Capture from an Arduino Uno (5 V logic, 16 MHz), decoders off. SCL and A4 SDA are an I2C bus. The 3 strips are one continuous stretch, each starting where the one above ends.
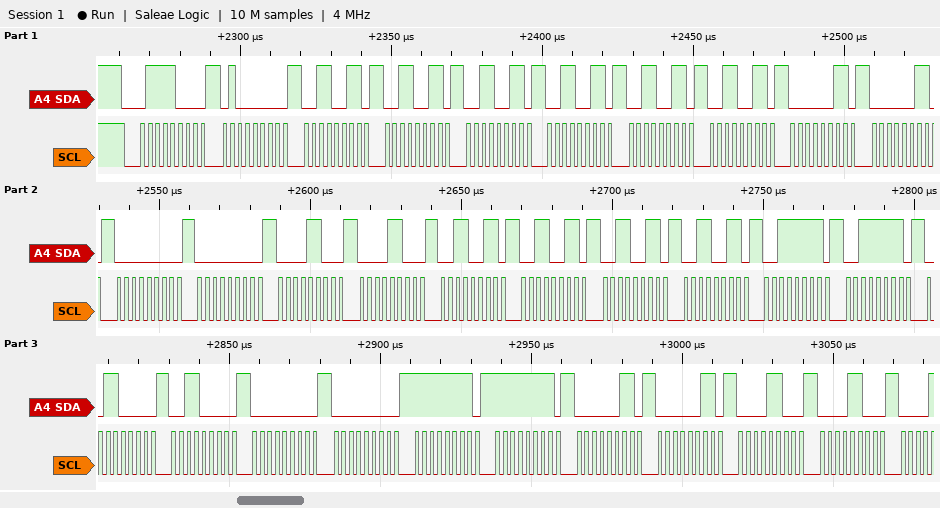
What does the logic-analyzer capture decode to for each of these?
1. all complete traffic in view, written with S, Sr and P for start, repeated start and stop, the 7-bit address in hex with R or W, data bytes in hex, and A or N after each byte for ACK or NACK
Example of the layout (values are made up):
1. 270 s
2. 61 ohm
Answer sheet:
1. S 3CW A 40 A 33 A 33 A 33 A 33 A 33 A 33 A 03 A 03 A 00 A 00 A 0C A 0C A 33 A 33 A 33 A 33 A 3F A 3F A 30 A 30 A 00 A 00 A FF A FF A 03 A 03 A 0C A 0C A
